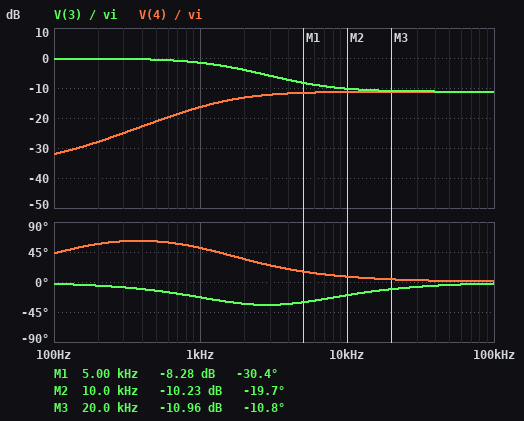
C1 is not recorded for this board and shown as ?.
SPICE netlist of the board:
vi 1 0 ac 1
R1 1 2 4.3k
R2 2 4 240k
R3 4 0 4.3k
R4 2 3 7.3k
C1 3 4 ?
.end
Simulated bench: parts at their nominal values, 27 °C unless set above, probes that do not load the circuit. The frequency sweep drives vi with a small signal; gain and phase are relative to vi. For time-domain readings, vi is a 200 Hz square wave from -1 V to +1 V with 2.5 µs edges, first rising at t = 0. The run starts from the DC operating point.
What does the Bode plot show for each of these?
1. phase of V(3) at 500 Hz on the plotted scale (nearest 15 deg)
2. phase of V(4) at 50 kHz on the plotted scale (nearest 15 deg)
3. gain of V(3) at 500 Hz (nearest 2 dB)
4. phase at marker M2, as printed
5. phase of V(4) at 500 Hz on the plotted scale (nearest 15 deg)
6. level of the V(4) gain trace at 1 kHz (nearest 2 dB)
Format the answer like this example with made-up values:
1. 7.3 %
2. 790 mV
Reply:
1. -15 deg
2. 0 deg
3. 0 dB
4. -19.7 deg
5. 60 deg
6. -16 dB
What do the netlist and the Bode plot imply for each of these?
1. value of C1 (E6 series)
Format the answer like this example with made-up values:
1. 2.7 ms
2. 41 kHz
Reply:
1. 6.8 nF
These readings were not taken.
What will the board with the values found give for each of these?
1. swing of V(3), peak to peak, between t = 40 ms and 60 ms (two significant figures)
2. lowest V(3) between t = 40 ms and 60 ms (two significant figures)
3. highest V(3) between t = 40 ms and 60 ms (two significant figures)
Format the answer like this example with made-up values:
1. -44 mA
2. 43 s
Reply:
1. 2.0 V
2. -980 mV
3. 980 mV
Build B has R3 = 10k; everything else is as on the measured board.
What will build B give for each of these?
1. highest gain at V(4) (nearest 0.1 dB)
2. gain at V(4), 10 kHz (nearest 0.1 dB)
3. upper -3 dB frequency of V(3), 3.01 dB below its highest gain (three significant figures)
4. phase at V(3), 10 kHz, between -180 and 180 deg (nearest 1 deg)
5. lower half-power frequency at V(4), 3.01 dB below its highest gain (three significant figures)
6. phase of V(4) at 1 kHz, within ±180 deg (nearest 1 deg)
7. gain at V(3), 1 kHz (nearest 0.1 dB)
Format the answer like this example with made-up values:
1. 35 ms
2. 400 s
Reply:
1. -6.6 dB
2. -6.7 dB
3. 1.52 kHz
4. -7 deg
5. 1.12 kHz
6. 43 deg
7. -2.0 dB
